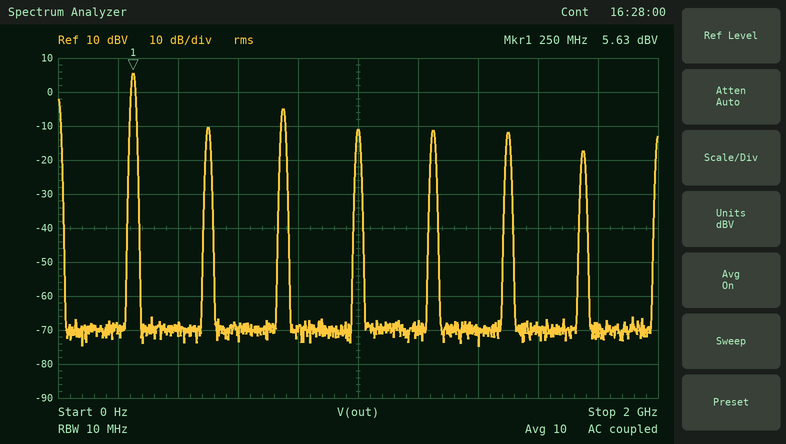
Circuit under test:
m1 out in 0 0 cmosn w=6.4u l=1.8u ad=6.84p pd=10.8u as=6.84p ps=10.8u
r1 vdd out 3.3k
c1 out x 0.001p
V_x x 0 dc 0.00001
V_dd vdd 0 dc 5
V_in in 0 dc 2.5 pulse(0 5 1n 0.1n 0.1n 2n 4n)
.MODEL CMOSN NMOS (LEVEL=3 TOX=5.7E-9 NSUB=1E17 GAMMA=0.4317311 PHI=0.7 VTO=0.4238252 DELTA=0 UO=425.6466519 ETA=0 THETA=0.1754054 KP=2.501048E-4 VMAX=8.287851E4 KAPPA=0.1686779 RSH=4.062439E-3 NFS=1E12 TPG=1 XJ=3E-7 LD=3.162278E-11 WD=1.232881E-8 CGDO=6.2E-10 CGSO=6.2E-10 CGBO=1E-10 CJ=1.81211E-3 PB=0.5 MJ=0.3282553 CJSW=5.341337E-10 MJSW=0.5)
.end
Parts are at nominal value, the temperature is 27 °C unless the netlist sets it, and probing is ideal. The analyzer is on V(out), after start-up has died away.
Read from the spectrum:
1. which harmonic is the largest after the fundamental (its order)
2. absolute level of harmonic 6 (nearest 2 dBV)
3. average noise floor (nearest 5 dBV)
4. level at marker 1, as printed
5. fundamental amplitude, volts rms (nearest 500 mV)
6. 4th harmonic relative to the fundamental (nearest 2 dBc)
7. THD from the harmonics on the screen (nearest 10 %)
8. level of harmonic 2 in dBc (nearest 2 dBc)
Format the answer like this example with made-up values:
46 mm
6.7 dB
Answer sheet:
3
-12 dBV
-70 dBV
5.63 dBV
2.0 V
-16 dBc
40 %
-16 dBc
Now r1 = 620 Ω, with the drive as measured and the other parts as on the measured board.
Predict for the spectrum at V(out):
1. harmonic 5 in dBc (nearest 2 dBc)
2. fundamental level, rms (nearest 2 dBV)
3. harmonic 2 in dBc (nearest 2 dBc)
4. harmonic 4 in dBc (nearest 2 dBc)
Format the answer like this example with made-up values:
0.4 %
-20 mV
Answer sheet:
-14 dBc
-2 dBV
-24 dBc
-24 dBc
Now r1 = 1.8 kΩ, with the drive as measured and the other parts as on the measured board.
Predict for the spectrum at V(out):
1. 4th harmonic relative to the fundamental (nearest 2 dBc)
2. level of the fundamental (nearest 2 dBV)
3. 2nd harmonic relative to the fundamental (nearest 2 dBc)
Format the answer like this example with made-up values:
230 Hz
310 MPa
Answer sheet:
-20 dBc
4 dBV
-20 dBc
